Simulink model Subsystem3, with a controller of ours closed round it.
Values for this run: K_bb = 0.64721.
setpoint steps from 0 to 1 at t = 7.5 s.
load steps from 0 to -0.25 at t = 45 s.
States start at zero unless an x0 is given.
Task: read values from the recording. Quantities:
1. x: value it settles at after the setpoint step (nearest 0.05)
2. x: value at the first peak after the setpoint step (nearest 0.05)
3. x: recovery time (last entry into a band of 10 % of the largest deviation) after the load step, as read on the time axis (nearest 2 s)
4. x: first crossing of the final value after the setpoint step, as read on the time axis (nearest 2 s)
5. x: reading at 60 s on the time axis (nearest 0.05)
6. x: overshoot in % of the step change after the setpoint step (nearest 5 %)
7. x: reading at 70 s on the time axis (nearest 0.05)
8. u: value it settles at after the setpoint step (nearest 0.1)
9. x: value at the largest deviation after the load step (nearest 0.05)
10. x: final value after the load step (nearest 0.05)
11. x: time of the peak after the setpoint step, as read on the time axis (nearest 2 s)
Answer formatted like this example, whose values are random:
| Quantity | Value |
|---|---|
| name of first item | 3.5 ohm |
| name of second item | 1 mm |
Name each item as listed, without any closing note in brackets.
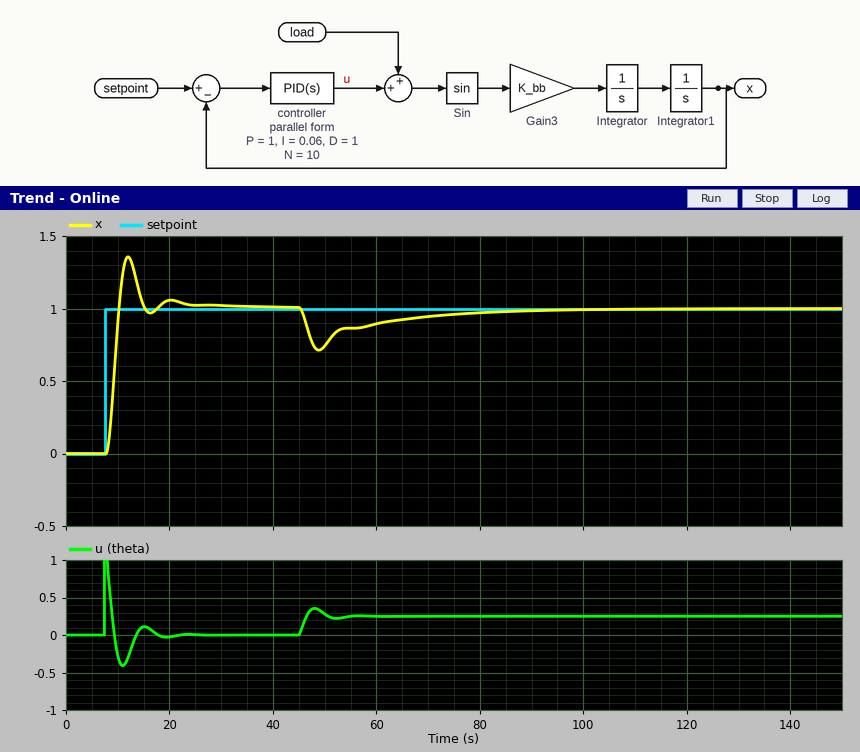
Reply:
| Quantity | Value |
|---|---|
| x: value it settles at after the setpoint step | 1.00 |
| x: value at the first peak after the setpoint step | 1.35 |
| x: recovery time (last entry into a band of 10 % of the largest deviation) after the load step, as read on the time axis | 80 s |
| x: first crossing of the final value after the setpoint step, as read on the time axis | 10 s |
| x: reading at 60 s on the time axis | 0.90 |
| x: overshoot in % of the step change after the setpoint step | 35 % |
| x: reading at 70 s on the time axis | 0.95 |
| u: value it settles at after the setpoint step | 0.0 |
| x: value at the largest deviation after the load step | 0.70 |
| x: final value after the load step | 1.00 |
| x: time of the peak after the setpoint step, as read on the time axis | 12 s |
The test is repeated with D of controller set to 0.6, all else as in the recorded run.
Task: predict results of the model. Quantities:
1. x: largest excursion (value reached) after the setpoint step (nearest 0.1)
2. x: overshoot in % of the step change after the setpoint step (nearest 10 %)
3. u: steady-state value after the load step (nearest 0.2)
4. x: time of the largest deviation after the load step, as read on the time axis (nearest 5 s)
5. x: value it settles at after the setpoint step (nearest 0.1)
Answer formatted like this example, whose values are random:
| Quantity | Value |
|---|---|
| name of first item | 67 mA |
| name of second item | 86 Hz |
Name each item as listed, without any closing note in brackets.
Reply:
| Quantity | Value |
|---|---|
| x: largest excursion (value reached) after the setpoint step | 1.6 |
| x: overshoot in % of the step change after the setpoint step | 60 % |
| u: steady-state value after the load step | 0.2 |
| x: time of the largest deviation after the load step, as read on the time axis | 50 s |
| x: value it settles at after the setpoint step | 1.0 |
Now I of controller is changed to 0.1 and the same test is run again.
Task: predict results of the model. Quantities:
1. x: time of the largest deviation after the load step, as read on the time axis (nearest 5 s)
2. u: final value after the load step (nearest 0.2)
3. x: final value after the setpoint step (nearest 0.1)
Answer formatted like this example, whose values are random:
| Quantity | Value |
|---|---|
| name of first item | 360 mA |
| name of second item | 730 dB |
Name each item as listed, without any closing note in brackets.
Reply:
| Quantity | Value |
|---|---|
| x: time of the largest deviation after the load step, as read on the time axis | 50 s |
| u: final value after the load step | 0.2 |
| x: final value after the setpoint step | 1.0 |
